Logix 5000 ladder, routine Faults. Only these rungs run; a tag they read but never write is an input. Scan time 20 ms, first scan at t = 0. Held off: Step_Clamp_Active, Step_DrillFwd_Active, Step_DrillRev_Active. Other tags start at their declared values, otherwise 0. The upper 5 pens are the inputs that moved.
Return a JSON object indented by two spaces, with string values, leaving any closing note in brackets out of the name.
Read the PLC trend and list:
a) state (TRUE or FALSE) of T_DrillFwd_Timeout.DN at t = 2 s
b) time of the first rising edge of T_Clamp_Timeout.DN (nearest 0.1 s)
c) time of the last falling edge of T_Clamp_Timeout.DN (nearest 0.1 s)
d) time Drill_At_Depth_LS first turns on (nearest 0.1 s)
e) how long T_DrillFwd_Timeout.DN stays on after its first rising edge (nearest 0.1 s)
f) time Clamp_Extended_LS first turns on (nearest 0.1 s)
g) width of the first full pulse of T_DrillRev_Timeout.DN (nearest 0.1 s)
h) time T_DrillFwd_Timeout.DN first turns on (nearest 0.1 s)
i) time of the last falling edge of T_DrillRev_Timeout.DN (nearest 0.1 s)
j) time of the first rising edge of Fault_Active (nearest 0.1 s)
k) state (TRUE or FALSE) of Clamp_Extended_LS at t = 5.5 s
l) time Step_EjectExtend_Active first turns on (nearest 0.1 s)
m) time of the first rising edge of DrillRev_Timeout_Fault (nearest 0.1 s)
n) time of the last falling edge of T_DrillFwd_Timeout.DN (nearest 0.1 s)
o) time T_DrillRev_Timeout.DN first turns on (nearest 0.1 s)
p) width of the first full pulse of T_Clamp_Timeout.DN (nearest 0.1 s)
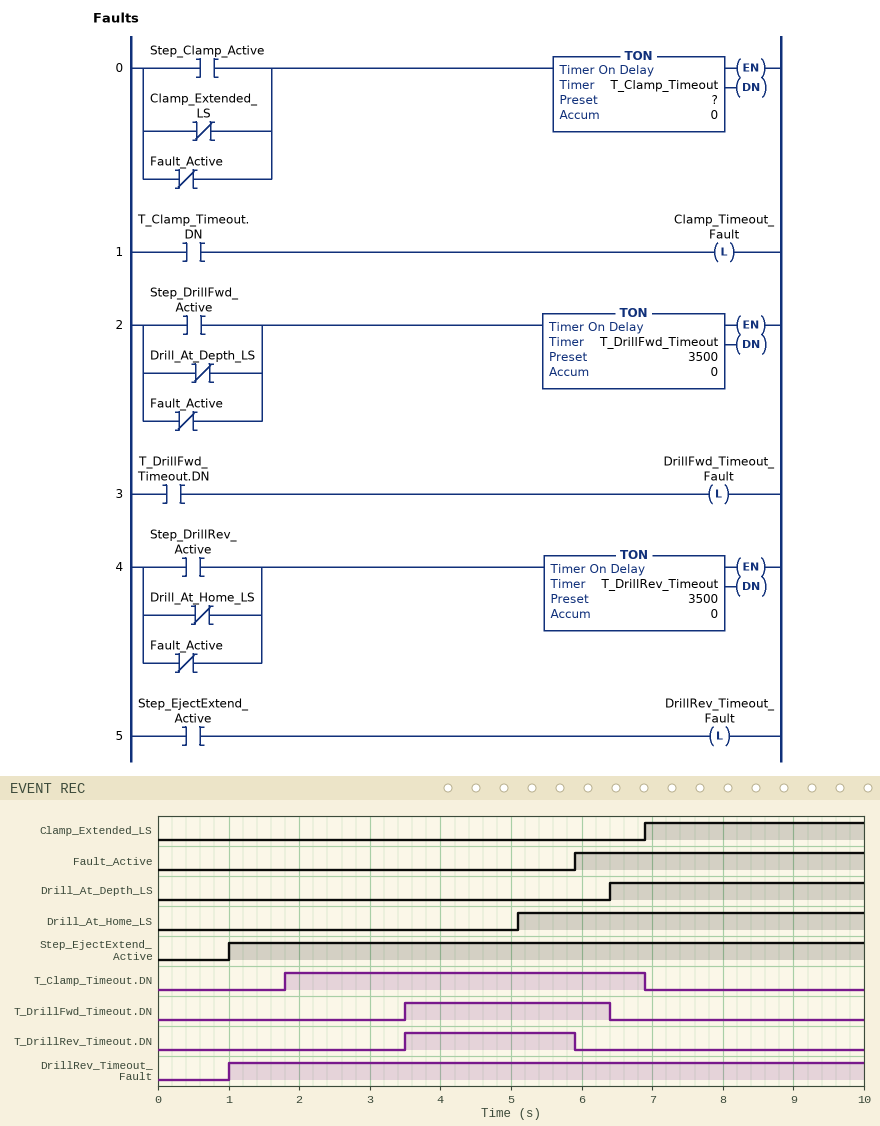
{
  "state (TRUE or FALSE) of T_DrillFwd_Timeout.DN at t = 2 s": "FALSE",
  "time of the first rising edge of T_Clamp_Timeout.DN": "1.8 s",
  "time of the last falling edge of T_Clamp_Timeout.DN": "6.9 s",
  "time Drill_At_Depth_LS first turns on": "6.4 s",
  "how long T_DrillFwd_Timeout.DN stays on after its first rising edge": "2.9 s",
  "time Clamp_Extended_LS first turns on": "6.9 s",
  "width of the first full pulse of T_DrillRev_Timeout.DN": "2.4 s",
  "time T_DrillFwd_Timeout.DN first turns on": "3.5 s",
  "time of the last falling edge of T_DrillRev_Timeout.DN": "5.9 s",
  "time of the first rising edge of Fault_Active": "5.9 s",
  "state (TRUE or FALSE) of Clamp_Extended_LS at t = 5.5 s": "FALSE",
  "time Step_EjectExtend_Active first turns on": "1.0 s",
  "time of the first rising edge of DrillRev_Timeout_Fault": "1.0 s",
  "time of the last falling edge of T_DrillFwd_Timeout.DN": "6.4 s",
  "time T_DrillRev_Timeout.DN first turns on": "3.5 s",
  "width of the first full pulse of T_Clamp_Timeout.DN": "5.1 s"
}
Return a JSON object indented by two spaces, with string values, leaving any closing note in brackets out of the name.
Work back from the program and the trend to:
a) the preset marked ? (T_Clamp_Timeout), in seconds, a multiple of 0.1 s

{
  "the preset marked ? (T_Clamp_Timeout), in seconds, a multiple of 0.1 s": "1.8 s"
}
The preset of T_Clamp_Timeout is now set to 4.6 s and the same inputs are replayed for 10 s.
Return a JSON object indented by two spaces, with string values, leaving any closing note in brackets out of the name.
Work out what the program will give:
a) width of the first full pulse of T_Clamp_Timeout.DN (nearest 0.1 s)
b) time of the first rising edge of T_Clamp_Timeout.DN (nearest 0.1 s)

{
  "width of the first full pulse of T_Clamp_Timeout.DN": "2.3 s",
  "time of the first rising edge of T_Clamp_Timeout.DN": "4.6 s"
}
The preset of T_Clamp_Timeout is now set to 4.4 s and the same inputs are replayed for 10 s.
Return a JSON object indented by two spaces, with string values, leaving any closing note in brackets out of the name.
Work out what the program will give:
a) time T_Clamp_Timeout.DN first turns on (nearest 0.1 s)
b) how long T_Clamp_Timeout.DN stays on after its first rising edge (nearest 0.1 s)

{
  "time T_Clamp_Timeout.DN first turns on": "4.4 s",
  "how long T_Clamp_Timeout.DN stays on after its first rising edge": "2.5 s"
}
